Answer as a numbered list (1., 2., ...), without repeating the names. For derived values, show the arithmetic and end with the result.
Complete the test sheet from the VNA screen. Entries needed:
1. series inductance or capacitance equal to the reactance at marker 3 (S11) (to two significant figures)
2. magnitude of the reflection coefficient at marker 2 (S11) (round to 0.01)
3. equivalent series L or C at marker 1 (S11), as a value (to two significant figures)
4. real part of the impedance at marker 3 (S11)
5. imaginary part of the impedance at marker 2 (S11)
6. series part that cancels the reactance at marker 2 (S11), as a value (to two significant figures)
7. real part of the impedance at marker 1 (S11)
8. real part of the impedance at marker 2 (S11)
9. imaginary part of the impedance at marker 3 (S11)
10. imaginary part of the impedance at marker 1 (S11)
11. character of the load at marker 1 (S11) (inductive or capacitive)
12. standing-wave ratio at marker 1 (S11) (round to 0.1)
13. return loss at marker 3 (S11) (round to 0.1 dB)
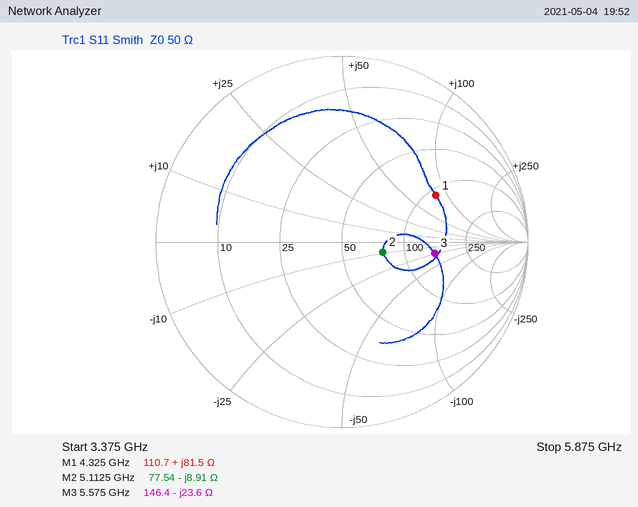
1. C = 1/(2π × 5.575 GHz × 23.6 Ω) ≈ 1.2 pF
2. 0.23
3. L = 81.5 Ω/(2π × 4.325 GHz) ≈ 3.0 nH
4. 146.4 Ω
5. -8.91 Ω
6. L = 8.91 Ω/(2π × 5.1125 GHz) ≈ 277 pH, so 280 pH to two significant figures
7. 110.7 Ω
8. 77.54 Ω
9. -23.6 Ω
10. +81.5 Ω
11. inductive
12. 3.6
13. 6.0 dB
